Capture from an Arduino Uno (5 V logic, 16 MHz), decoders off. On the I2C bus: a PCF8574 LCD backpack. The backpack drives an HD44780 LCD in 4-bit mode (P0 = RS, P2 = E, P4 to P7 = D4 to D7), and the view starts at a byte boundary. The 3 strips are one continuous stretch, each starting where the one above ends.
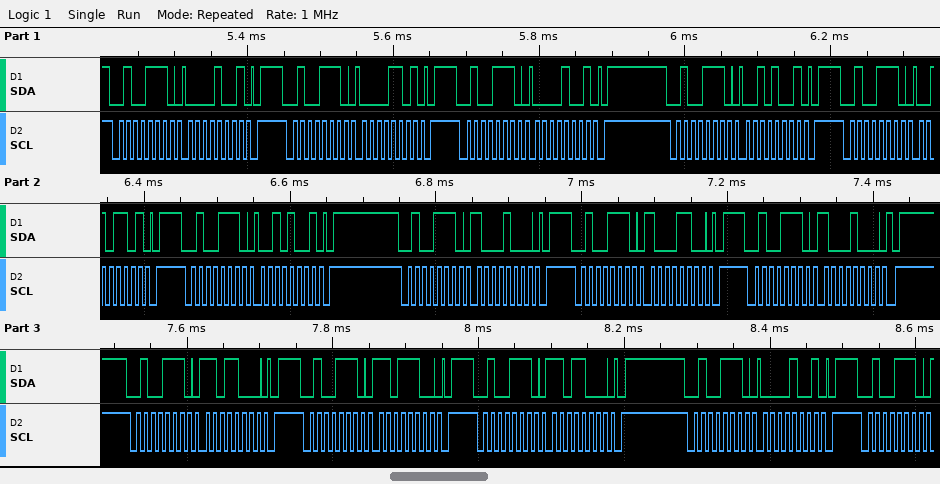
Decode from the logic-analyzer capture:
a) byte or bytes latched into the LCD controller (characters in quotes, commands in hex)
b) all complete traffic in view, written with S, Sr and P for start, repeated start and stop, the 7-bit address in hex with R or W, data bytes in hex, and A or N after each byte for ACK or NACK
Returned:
data 0x02 0x8D
S 27W A 09 A P S 27W A 0D A P S 27W A 09 A P S 27W A 29 A P S 27W A 2D A P S 27W A 29 A P S 27W A 88 A P S 27W A 8C A P S 27W A 88 A P S 27W A D8 A P S 27W A DC A P S 27W A D8 A P S 27W A 09 A P S 27W A
